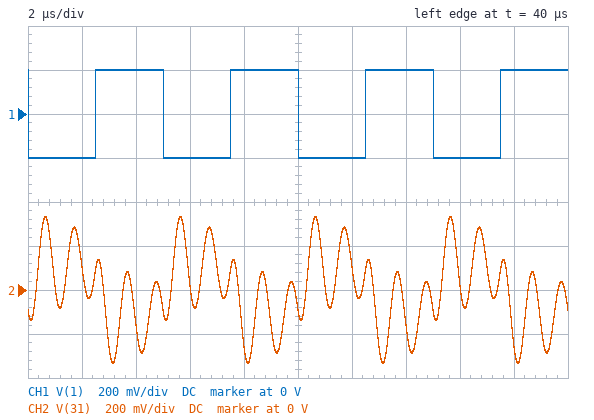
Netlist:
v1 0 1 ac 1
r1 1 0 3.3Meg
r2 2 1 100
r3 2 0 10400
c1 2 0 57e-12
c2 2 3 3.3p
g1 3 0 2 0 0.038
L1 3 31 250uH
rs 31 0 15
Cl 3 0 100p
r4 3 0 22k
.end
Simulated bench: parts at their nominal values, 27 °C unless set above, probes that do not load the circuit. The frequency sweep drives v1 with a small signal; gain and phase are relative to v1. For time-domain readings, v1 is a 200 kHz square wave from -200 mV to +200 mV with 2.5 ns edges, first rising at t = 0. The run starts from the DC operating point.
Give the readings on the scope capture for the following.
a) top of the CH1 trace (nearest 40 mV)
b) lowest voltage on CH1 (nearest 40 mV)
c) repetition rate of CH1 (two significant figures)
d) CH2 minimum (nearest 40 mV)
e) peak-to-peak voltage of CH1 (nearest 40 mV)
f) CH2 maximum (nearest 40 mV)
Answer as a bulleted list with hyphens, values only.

- 200 mV
- -200 mV
- 200 kHz
- -320 mV
- 400 mV
- 320 mV
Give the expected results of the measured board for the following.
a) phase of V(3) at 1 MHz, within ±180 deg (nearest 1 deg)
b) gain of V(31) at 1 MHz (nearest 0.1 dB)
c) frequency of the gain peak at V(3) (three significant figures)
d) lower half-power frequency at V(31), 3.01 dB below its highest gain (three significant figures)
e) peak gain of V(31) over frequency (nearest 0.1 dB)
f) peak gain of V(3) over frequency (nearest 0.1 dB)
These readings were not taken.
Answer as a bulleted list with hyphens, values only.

- -61 deg
- 10.6 dB
- 936 kHz
- 896 kHz
- 16.9 dB
- 56.7 dB
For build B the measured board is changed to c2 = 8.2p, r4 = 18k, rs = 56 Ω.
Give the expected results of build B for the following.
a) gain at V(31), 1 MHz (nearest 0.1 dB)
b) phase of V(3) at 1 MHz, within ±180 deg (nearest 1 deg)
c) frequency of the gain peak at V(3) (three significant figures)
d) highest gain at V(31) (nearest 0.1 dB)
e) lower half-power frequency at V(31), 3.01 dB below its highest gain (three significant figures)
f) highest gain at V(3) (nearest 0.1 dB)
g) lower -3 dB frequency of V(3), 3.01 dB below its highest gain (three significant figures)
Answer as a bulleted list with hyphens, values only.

- 14.5 dB
- -72 deg
- 855 kHz
- 24.6 dB
- 797 kHz
- 52.2 dB
- 803 kHz
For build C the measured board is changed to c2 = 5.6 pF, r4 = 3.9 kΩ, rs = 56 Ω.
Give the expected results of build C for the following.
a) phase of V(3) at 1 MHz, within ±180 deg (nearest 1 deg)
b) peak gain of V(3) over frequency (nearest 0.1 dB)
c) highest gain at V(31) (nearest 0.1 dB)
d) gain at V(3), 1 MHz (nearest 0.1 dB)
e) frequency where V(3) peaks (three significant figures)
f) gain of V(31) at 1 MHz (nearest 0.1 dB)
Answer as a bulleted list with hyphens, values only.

- -32 deg
- 42.3 dB
- 14.4 dB
- 41.2 dB
- 900 kHz
- 12.3 dB
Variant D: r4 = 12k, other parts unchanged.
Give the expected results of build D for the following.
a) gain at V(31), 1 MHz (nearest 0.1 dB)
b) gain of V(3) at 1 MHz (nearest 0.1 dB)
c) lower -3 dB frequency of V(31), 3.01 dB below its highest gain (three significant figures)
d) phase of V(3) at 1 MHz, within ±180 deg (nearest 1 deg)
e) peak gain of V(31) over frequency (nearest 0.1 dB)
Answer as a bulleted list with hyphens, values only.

- 8.9 dB
- 49.3 dB
- 865 kHz
- -47 deg
- 12.3 dB
